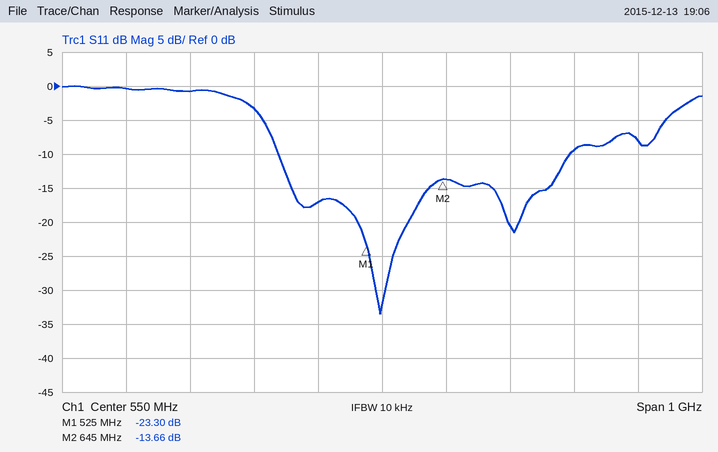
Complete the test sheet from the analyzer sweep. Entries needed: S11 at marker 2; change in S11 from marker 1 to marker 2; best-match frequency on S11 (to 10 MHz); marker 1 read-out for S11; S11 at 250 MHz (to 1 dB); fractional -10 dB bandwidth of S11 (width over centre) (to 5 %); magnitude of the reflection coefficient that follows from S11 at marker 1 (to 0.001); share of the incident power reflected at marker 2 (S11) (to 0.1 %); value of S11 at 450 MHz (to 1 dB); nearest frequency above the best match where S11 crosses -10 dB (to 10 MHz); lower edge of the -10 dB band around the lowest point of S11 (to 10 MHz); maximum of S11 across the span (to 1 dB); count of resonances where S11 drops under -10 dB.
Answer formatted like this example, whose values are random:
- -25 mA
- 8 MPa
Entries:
- -13.66 dB
- 9.64 dB
- 550 MHz
- -23.30 dB
- -1 dB
- 75 %
- 0.068
- 4.3 %
- -17 dB
- 840 MHz
- 390 MHz
- 0 dB
- 2
